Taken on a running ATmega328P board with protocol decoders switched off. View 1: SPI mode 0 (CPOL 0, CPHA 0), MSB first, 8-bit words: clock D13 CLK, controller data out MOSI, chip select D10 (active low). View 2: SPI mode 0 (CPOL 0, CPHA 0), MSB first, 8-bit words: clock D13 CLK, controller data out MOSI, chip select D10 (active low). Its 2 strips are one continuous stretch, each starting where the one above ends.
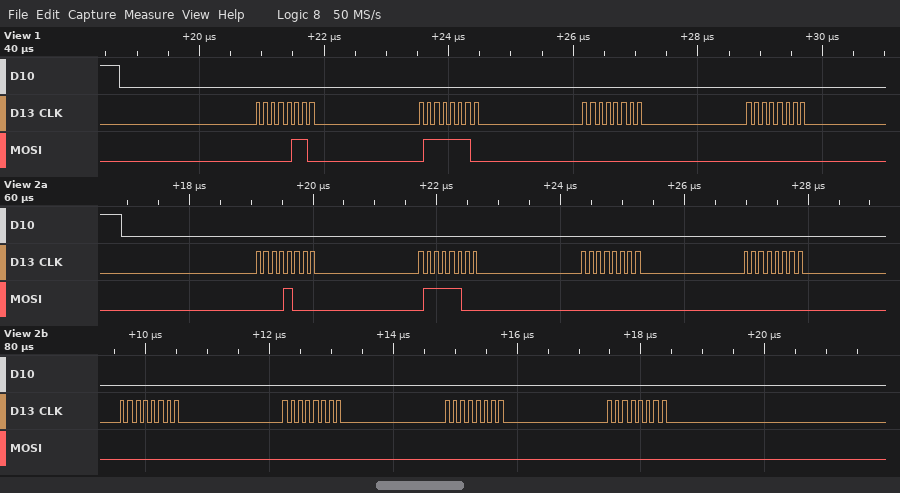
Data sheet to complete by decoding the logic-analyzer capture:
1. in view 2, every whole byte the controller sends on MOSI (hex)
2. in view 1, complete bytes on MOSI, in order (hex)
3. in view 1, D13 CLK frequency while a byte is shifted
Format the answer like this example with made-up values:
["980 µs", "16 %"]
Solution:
["08 7C 00 00 00 00 00 00", "06 7E 00 00", "8 MHz"]
